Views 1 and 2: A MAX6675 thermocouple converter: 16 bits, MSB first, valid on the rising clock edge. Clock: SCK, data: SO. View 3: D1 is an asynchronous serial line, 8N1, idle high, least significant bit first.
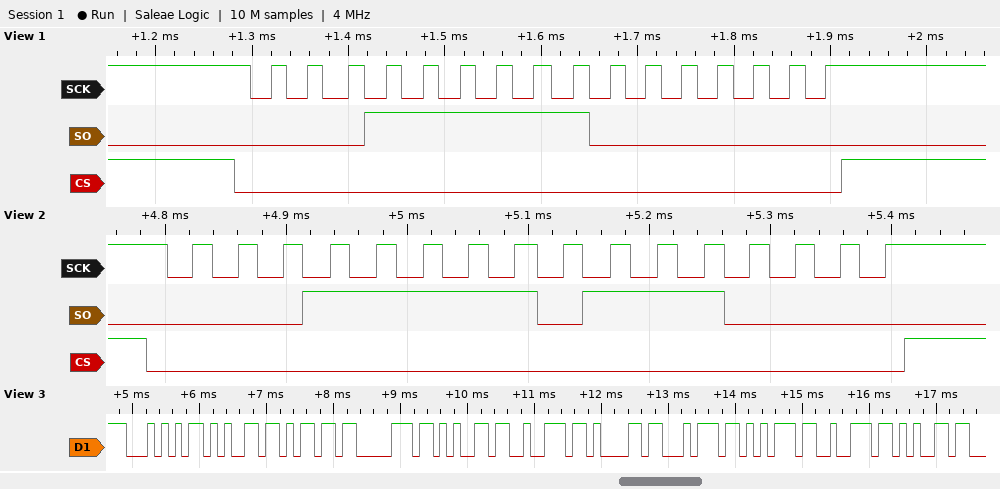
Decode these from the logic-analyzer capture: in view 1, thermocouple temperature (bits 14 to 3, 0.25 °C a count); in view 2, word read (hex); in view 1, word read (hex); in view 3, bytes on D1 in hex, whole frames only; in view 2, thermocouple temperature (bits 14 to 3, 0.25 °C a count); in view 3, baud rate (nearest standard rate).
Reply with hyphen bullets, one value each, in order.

- 252.00 °C
- 0x1F70
- 0x1F80
- 54 65 6D 70 65 72 61 74 75 72 65
- 251.50 °C
- 9600 baud
